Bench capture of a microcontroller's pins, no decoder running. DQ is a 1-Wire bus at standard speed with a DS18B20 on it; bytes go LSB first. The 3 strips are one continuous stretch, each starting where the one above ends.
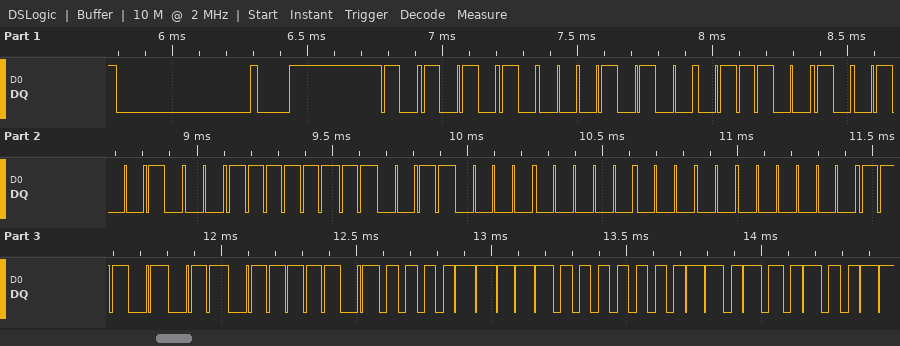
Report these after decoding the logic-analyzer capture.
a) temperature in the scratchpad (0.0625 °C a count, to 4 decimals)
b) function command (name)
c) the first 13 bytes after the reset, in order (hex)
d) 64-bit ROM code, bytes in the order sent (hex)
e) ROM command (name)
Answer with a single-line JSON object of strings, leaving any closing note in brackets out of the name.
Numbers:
{"temperature in the scratchpad": "31.0000 °C", "function command": "Read Scratchpad", "the first 13 bytes after the reset, in order": "55 28 4E 12 FF 0C 00 00 D7 BE F0 01 4B", "64-bit ROM code, bytes in the order sent": "28 4E 12 FF 0C 00 00 D7", "ROM command": "Match ROM"}
